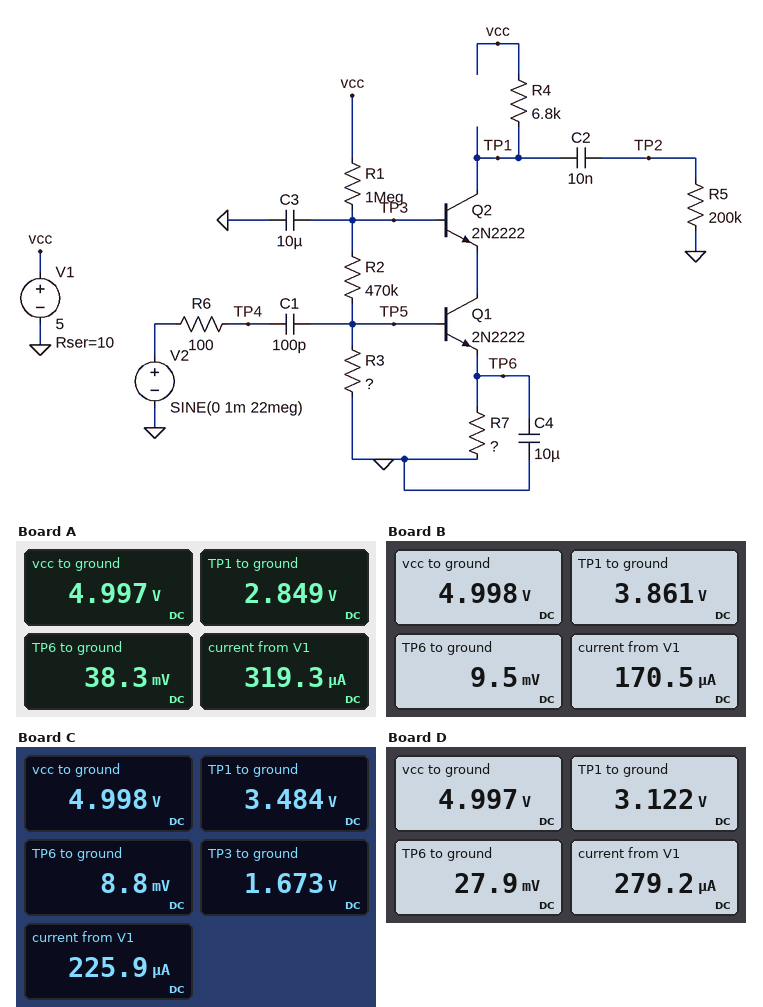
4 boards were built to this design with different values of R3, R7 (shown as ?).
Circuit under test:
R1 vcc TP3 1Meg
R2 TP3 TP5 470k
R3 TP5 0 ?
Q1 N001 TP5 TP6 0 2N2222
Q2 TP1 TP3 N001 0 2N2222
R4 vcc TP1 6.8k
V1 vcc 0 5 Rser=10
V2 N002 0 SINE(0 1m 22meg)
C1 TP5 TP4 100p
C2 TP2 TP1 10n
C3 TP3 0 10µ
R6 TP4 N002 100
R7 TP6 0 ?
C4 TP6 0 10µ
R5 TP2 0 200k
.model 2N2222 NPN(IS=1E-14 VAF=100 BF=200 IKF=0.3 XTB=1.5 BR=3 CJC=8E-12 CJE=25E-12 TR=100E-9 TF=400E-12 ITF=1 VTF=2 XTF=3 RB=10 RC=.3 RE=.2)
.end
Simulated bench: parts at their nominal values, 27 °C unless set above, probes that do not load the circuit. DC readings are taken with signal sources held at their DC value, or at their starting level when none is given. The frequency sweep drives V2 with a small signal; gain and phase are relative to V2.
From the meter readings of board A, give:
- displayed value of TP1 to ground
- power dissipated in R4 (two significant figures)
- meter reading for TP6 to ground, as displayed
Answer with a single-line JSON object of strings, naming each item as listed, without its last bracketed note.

{"displayed value of TP1 to ground": "2.849 V", "power dissipated in R4": "680 µW", "meter reading for TP6 to ground, as displayed": "38.3 mV"}
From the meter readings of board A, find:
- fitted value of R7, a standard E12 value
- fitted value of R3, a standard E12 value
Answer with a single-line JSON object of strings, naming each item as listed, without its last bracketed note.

{"fitted value of R7, a standard E12 value": "120 Ω", "fitted value of R3, a standard E12 value": "2.2 MΩ"}
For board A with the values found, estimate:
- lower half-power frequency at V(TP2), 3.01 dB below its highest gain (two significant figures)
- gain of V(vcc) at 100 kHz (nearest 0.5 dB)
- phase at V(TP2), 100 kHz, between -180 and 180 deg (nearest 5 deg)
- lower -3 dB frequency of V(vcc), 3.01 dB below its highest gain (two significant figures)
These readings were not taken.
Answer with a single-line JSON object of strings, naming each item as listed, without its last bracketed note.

{"lower half-power frequency at V(TP2), 3.01 dB below its highest gain": "62 kHz", "gain of V(vcc) at 100 kHz": "-24.0 dB", "phase at V(TP2), 100 kHz, between -180 and 180 deg": "-150 deg", "lower -3 dB frequency of V(vcc), 3.01 dB below its highest gain": "62 kHz"}
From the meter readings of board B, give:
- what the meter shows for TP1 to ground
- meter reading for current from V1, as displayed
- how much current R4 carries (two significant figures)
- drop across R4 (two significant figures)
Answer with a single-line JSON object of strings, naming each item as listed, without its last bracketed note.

{"what the meter shows for TP1 to ground": "3.861 V", "meter reading for current from V1, as displayed": "170.5 µA", "how much current R4 carries": "170 µA", "drop across R4": "1.1 V"}
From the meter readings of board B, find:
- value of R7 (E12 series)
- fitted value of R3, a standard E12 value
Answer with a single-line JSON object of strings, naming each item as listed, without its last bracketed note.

{"value of R7": "56 Ω", "fitted value of R3, a standard E12 value": "390 kΩ"}
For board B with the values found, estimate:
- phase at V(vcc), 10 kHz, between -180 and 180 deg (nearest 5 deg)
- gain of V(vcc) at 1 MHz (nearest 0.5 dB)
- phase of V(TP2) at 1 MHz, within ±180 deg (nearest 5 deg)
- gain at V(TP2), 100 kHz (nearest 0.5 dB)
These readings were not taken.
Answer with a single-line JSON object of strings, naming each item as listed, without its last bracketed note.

{"phase at V(vcc), 10 kHz, between -180 and 180 deg": "-105 deg", "gain of V(vcc) at 1 MHz": "-28.0 dB", "phase of V(TP2) at 1 MHz, within ±180 deg": "165 deg", "gain at V(TP2), 100 kHz": "28.0 dB"}
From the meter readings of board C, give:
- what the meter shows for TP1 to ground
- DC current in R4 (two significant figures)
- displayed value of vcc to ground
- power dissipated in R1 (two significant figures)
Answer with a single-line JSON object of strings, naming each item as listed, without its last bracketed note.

{"what the meter shows for TP1 to ground": "3.484 V", "DC current in R4": "220 µA", "displayed value of vcc to ground": "4.998 V", "power dissipated in R1": "11 µW"}
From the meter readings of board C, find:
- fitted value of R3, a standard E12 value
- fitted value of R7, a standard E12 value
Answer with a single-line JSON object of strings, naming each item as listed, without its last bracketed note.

{"fitted value of R3, a standard E12 value": "560 kΩ", "fitted value of R7, a standard E12 value": "39 Ω"}
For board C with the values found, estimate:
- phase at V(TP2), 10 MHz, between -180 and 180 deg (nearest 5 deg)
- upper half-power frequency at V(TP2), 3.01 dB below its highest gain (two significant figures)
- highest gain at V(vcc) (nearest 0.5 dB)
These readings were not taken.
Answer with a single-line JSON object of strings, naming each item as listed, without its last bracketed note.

{"phase at V(TP2), 10 MHz, between -180 and 180 deg": "80 deg", "upper half-power frequency at V(TP2), 3.01 dB below its highest gain": "4.4 MHz", "highest gain at V(vcc)": "-25.5 dB"}
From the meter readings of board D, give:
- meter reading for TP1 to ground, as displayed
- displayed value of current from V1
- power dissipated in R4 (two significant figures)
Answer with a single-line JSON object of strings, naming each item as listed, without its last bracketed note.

{"meter reading for TP1 to ground, as displayed": "3.122 V", "displayed value of current from V1": "279.2 µA", "power dissipated in R4": "520 µW"}
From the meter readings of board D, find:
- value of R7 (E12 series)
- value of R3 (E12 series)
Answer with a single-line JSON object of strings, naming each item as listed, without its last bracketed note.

{"value of R7": "100 Ω", "value of R3": "1 MΩ"}
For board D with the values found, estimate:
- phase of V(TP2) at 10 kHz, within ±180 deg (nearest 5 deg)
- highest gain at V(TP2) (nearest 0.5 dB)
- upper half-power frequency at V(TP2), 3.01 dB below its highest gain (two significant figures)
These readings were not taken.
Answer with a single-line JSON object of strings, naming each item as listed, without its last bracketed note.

{"phase of V(TP2) at 10 kHz, within ±180 deg": "-100 deg", "highest gain at V(TP2)": "33.0 dB", "upper half-power frequency at V(TP2), 3.01 dB below its highest gain": "4.3 MHz"}
